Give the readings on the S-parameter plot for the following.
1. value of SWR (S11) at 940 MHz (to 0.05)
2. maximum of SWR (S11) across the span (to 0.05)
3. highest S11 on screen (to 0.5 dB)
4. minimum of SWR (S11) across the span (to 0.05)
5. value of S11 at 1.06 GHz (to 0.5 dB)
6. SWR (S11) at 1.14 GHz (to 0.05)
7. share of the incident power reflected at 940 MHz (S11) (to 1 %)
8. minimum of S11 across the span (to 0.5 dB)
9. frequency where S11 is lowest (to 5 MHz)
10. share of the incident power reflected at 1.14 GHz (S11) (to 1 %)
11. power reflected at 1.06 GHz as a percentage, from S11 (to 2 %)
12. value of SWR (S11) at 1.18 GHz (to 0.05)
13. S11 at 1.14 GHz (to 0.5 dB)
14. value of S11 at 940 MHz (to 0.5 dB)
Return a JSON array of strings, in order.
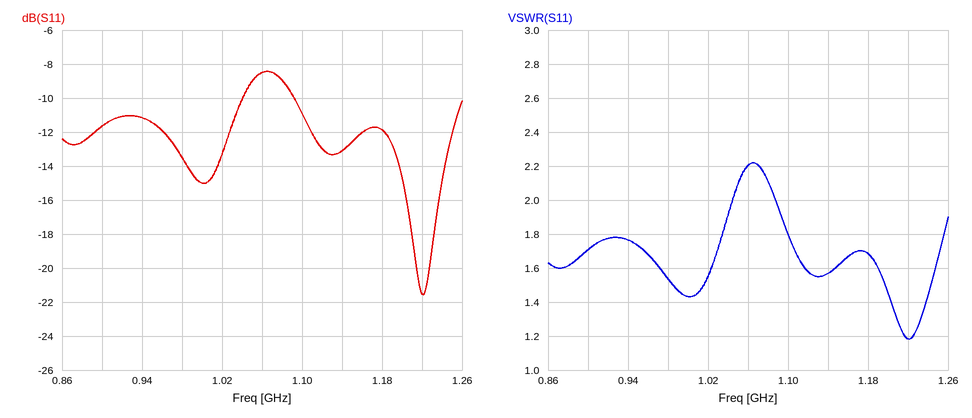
["1.75", "2.20", "-8.5 dB", "1.20", "-8.5 dB", "1.55", "8 %", "-21.5 dB", "1.220 GHz", "5 %", "14 %", "1.70", "-13.0 dB", "-11.0 dB"]
